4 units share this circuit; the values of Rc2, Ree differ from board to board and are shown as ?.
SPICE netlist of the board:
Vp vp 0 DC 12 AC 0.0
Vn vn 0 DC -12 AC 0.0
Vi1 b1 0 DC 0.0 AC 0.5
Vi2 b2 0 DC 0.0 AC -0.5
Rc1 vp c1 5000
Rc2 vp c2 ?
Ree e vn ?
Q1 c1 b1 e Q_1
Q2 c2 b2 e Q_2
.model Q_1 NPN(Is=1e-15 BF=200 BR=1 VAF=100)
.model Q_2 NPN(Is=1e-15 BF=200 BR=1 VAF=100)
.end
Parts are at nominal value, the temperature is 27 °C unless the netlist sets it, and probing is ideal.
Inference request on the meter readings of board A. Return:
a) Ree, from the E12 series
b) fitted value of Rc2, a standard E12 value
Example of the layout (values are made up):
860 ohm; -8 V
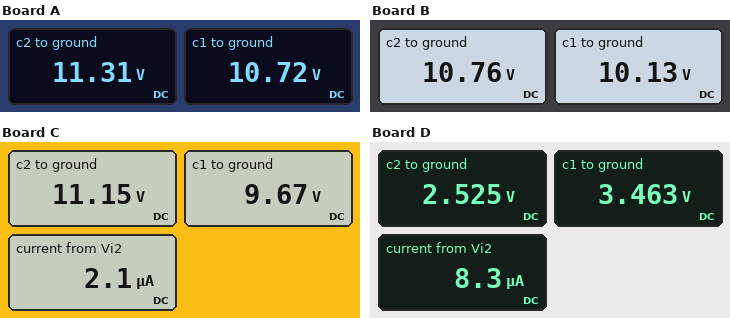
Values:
22 kΩ; 2.7 kΩ
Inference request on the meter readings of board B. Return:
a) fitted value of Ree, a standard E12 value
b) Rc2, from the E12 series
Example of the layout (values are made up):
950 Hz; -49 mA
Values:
15 kΩ; 3.3 kΩ
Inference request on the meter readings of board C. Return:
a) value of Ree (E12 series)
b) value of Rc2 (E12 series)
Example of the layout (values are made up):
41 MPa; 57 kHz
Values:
12 kΩ; 1.8 kΩ
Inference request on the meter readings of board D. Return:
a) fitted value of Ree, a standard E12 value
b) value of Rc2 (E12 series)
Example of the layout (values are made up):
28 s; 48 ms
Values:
3.3 kΩ; 5.6 kΩ
